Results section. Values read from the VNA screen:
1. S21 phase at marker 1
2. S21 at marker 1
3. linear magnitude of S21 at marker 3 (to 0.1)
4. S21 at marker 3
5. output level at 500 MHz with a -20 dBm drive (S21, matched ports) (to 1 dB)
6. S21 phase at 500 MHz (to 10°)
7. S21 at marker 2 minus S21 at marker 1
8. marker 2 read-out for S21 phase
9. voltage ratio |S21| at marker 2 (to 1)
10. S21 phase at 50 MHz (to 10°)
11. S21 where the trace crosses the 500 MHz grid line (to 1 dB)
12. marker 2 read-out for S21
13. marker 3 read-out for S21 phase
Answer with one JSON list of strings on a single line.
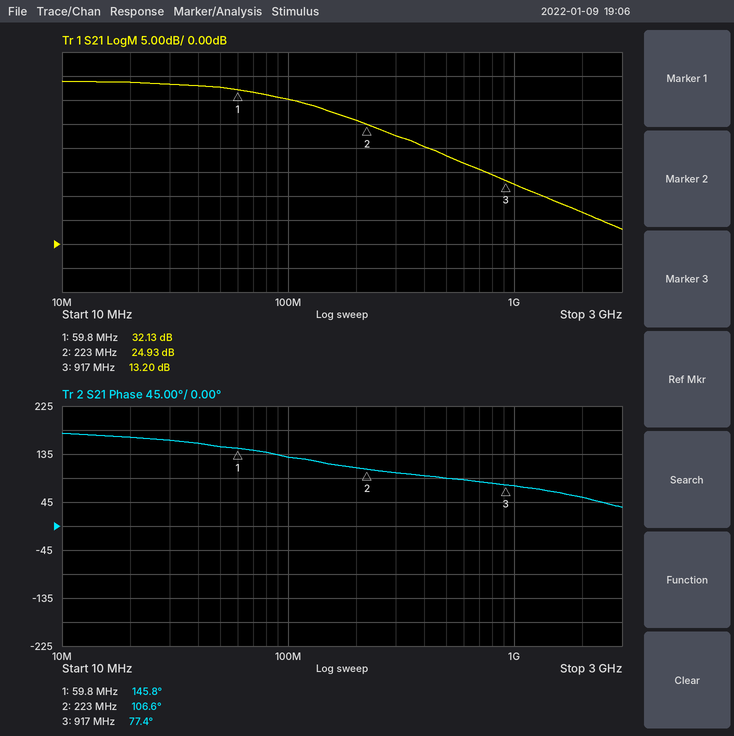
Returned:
["145.8°", "32.13 dB", "4.6", "13.20 dB", "-2 dBm", "90°", "-7.20 dB", "106.6°", "18", "150°", "18 dB", "24.93 dB", "77.4°"]
